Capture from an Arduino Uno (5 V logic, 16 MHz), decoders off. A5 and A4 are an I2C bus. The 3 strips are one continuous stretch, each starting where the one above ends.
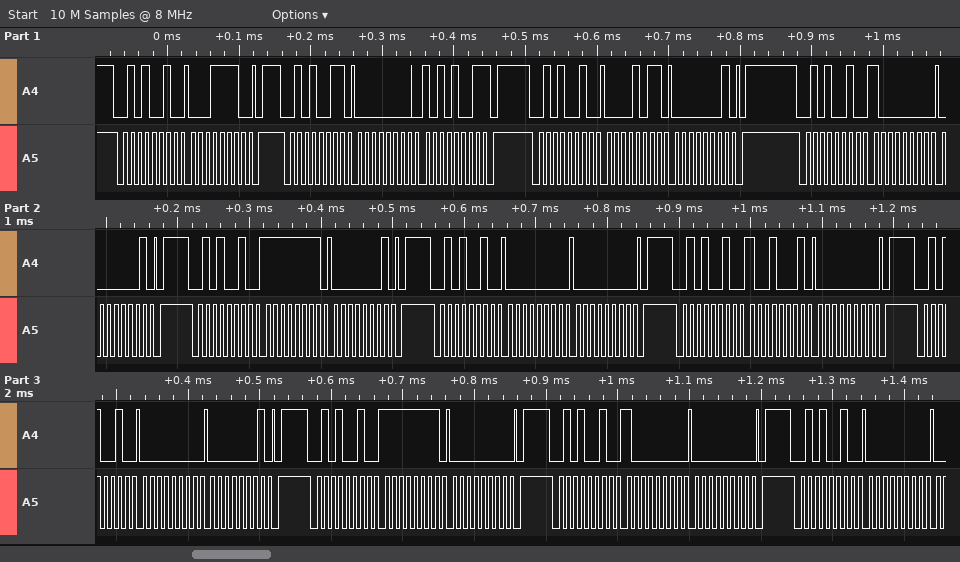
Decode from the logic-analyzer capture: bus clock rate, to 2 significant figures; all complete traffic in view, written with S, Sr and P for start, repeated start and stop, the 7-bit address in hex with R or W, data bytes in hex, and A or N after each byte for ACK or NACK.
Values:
100 kHz
S 29W A 1E A P S 29R A 00 A A9 N P S 29W A 0B A 01 A P S 29W A 80 A 01 A P S 29W A FF A 01 A P S 29W A 00 A 00 A P S 29W A 91 A 00 A P S 29W A 00 A 01 A P S 29W A FF A 00 A P S 29W A 80 A 00 A P S 29W A 00 A
